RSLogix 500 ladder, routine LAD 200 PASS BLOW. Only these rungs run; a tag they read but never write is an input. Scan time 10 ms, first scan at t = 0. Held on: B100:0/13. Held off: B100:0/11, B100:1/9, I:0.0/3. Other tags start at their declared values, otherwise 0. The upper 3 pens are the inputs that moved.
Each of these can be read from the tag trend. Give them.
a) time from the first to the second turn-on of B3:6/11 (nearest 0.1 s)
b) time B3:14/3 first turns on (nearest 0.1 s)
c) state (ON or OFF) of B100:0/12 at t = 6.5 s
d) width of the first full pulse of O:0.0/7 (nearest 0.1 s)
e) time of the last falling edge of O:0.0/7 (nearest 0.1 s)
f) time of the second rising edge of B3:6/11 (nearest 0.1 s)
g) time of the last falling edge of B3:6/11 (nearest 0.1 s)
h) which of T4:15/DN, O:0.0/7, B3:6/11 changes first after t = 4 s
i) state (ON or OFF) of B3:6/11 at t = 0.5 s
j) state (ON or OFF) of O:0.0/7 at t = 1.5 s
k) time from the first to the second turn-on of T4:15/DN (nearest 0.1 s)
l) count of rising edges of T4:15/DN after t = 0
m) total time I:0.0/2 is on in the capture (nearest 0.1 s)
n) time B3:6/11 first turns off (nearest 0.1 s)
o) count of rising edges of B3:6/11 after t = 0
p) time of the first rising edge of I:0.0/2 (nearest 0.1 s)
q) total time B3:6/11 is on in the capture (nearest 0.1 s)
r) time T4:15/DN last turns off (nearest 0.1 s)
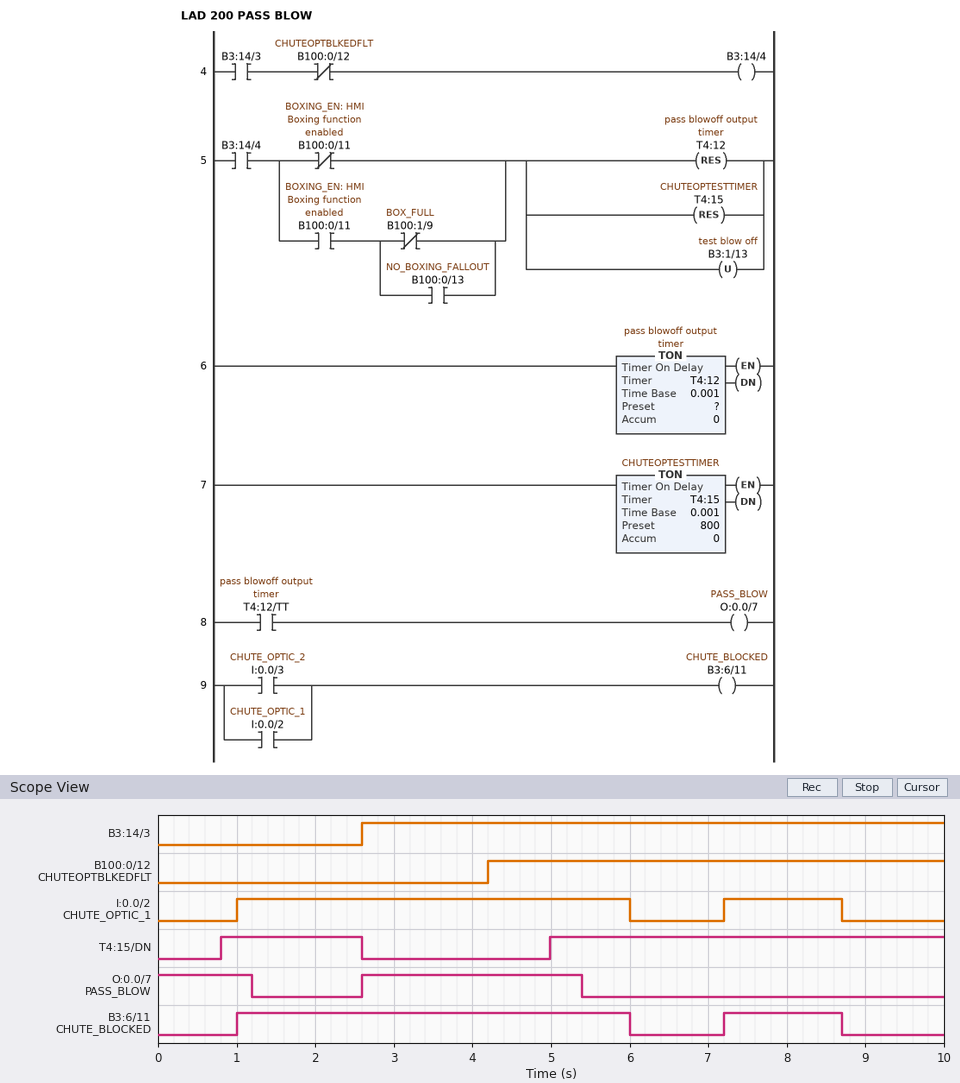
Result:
6.2 s
2.6 s
ON
2.8 s
5.4 s
7.2 s
8.7 s
T4:15/DN
OFF
OFF
4.2 s
2
6.5 s
6.0 s
2
1.0 s
6.5 s
2.6 s
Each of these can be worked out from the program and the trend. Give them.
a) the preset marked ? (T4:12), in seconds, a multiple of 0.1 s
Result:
1.2 s
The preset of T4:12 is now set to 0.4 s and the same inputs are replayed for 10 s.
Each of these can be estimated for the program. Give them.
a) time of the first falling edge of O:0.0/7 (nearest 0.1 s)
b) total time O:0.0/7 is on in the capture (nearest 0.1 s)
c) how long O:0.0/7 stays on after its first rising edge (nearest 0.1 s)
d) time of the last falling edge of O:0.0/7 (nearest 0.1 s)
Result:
0.4 s
2.4 s
2.0 s
4.6 s
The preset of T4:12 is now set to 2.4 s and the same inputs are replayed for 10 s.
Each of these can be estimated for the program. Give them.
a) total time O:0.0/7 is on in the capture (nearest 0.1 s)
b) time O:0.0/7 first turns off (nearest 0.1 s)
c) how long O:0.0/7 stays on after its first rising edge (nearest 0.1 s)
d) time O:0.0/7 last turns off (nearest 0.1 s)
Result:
6.4 s
2.4 s
4.0 s
6.6 s
